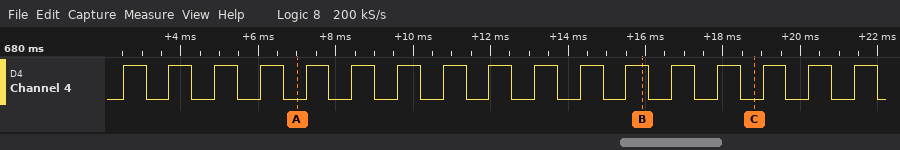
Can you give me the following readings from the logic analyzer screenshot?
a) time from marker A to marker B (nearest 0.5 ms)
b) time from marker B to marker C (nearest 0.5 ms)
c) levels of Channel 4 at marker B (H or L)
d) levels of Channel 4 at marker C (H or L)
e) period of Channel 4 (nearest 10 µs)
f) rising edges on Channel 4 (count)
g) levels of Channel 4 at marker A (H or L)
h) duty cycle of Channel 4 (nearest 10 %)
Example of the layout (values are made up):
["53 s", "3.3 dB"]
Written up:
["9 ms", "3 ms", "Channel 4=H", "Channel 4=L", "1180 µs", "17", "Channel 4=L", "50 %"]
